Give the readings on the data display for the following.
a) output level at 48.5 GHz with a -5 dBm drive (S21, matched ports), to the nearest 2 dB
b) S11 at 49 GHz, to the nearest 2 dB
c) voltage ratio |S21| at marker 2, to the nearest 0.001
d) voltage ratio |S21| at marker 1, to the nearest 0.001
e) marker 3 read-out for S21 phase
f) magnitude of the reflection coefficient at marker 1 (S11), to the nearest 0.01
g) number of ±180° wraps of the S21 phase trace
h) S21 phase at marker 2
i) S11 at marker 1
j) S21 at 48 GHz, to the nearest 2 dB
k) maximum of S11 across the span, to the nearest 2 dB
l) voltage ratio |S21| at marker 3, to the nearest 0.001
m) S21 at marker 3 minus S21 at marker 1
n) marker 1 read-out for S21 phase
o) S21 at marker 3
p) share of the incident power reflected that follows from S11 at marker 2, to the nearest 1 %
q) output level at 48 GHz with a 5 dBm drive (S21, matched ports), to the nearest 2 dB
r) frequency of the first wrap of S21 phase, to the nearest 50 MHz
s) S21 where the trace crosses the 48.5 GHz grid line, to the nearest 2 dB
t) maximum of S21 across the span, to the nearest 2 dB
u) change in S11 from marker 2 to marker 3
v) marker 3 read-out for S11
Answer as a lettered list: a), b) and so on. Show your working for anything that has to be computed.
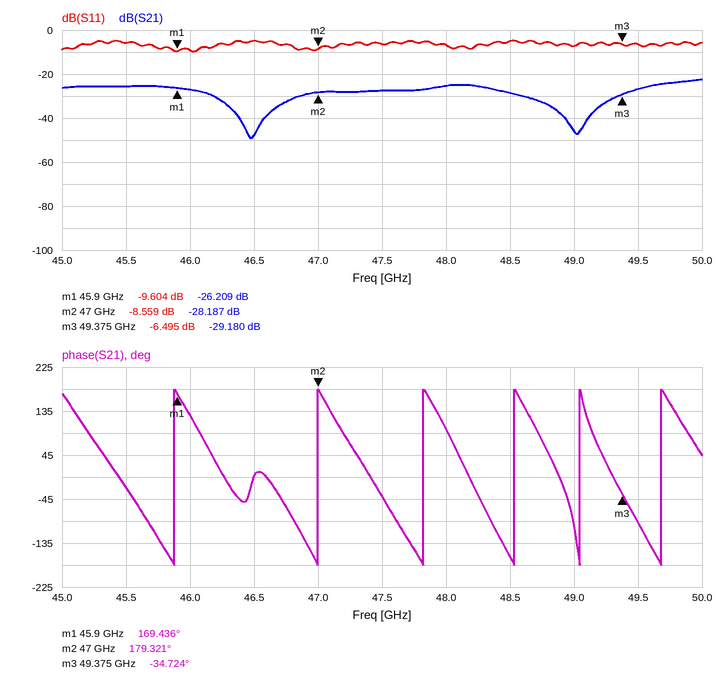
a) -5 dBm + (-28 dB) = -34 dBm
b) -8 dB
c) 10^(-28.187/20) ≈ 0.039
d) 10^(-26.209/20) ≈ 0.049
e) -34.724°
f) 10^(-9.604/20) ≈ 0.33
g) 6
h) 179.321°
i) -9.604 dB
j) -26 dB
k) -4 dB
l) 10^(-29.18/20) ≈ 0.035
m) -29.18 − (-26.209) = -2.971 dB
n) 169.436°
o) -29.180 dB
p) 10^(-8.559/10) ≈ 14 %
q) 5 dBm + (-26 dB) = -20 dBm
r) 45.90 GHz
s) -28 dB
t) -22 dB
u) -6.495 − (-8.559) = 2.064 dB
v) -6.495 dB
